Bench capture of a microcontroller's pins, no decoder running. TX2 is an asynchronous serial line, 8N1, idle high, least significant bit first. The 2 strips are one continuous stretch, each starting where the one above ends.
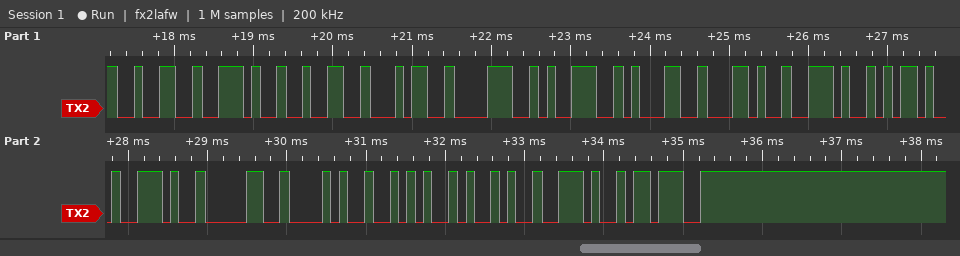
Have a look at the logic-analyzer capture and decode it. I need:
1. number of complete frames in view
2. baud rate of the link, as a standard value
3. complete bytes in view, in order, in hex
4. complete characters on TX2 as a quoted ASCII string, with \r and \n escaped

17
9600 baud
0x32 0x2E 0x32 0x34 0x38 0x39 0x31 0x2C 0x2E 0x2D 0x2E 0x30 0x28 0x2A 0x29 0x2E 0x3B
"2.24891,.-.0(*).;"
